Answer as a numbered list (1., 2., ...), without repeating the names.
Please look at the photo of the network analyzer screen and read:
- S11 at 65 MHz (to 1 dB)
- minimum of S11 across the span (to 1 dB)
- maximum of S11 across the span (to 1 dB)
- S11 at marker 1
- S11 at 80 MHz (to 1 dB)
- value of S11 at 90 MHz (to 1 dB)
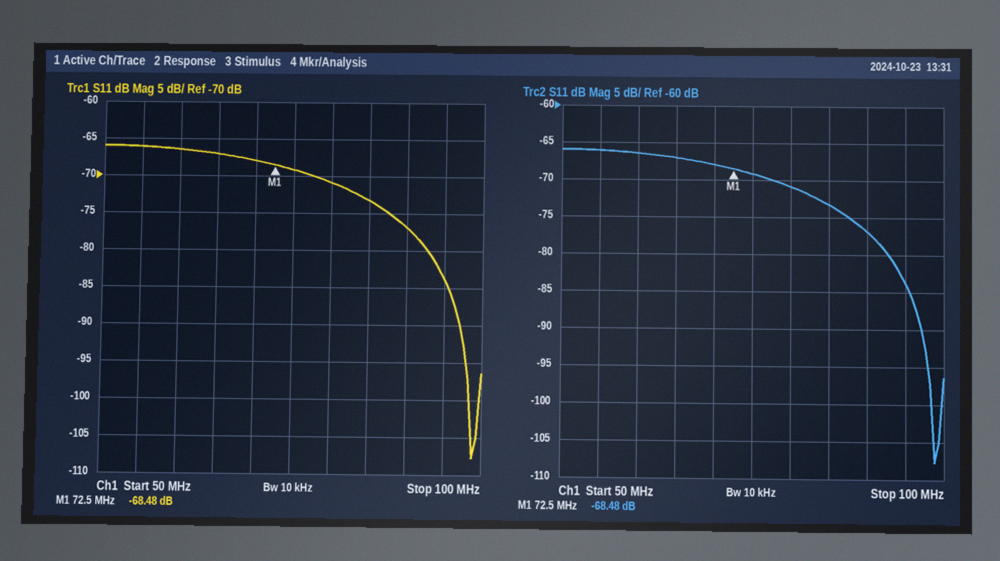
1. -67 dB
2. -108 dB
3. -66 dB
4. -68.48 dB
5. -71 dB
6. -77 dB
